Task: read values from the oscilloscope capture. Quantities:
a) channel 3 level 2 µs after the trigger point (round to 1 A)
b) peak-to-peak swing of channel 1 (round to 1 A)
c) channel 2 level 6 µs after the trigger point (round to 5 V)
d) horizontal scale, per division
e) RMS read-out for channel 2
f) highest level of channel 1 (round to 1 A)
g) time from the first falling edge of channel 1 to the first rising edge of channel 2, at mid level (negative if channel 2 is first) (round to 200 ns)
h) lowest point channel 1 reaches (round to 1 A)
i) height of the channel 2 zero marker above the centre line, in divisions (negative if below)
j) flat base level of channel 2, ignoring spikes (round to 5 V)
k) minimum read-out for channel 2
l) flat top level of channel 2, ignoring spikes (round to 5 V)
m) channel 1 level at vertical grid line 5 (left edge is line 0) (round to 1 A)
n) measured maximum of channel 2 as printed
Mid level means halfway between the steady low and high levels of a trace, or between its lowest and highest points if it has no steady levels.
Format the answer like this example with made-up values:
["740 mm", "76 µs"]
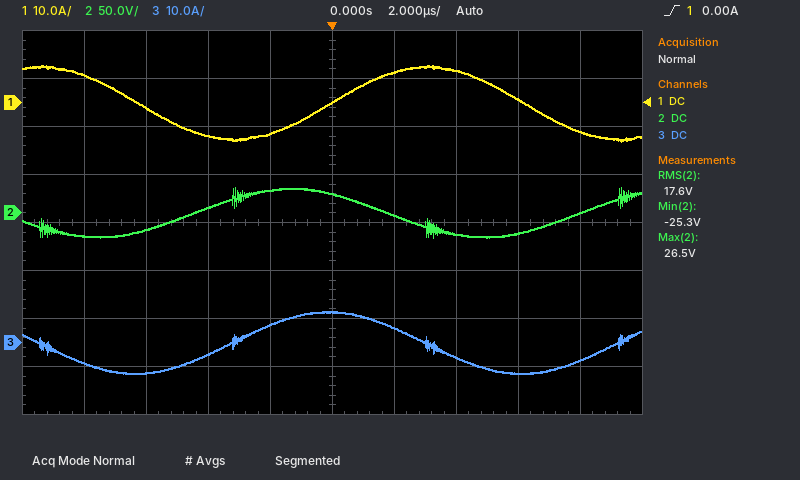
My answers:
["3 A", "16 A", "-20 V", "2 µs", "17.6 V", "8 A", "+1.8 µs", "-8 A", "+0.2 div", "-25 V", "-25.3 V", "25 V", "0 A", "26.5 V"]
